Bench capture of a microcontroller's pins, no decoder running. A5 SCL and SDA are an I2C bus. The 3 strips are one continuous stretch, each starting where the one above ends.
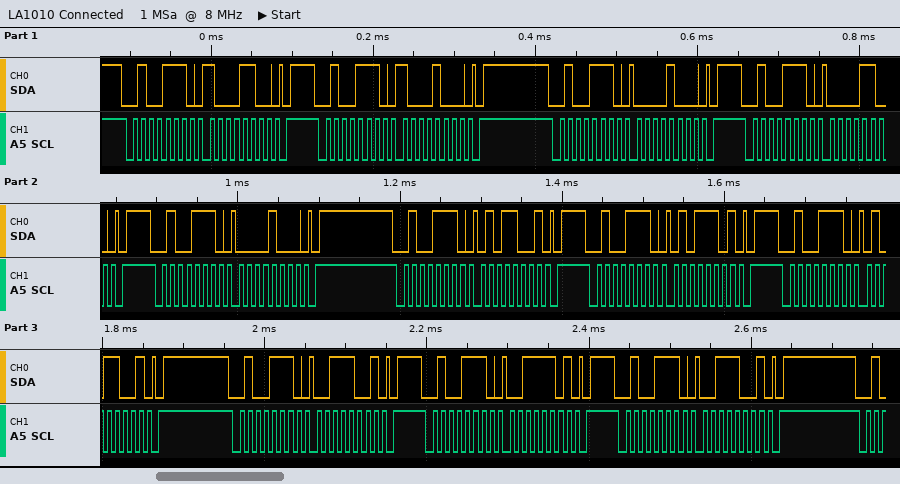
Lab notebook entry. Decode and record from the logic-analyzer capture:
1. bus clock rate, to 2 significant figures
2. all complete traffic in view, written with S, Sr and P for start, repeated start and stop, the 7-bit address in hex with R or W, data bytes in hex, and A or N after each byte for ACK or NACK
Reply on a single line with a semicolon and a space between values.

100 kHz; S 27W A 8C A P S 27W A 88 A P S 27W A 08 A P S 27W A 0C A P S 27W A 08 A P S 27W A 59 A P S 27W A 5D A P S 27W A 59 A P S 27W A 39 A P S 27W A 3D A P S 27W A 39 A P
